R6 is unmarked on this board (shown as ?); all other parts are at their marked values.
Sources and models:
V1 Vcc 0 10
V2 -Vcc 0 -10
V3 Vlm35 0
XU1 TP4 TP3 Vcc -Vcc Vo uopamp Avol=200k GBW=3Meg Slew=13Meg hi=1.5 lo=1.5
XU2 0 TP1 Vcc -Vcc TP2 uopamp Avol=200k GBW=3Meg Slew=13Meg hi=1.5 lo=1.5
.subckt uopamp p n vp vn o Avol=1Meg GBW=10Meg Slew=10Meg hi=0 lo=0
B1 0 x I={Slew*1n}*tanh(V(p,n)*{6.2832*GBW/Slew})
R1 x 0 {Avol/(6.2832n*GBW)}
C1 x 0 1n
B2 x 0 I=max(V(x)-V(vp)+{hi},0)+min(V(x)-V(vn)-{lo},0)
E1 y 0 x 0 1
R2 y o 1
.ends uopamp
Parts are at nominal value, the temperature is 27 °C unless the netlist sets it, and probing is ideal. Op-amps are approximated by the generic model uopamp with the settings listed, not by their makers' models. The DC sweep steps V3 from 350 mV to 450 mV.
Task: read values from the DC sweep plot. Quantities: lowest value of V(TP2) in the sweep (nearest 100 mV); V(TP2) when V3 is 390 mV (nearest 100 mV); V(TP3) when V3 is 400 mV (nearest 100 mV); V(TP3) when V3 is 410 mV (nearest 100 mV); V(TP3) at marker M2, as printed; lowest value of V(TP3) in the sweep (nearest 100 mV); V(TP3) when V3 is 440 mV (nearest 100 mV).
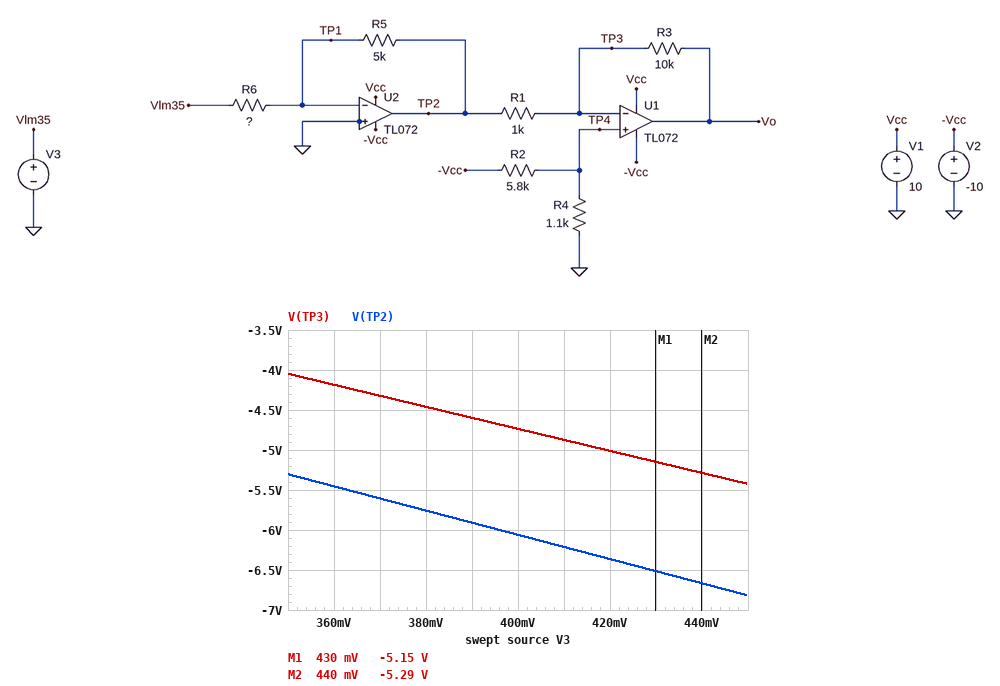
-6.8 V
-5.9 V
-4.7 V
-4.9 V
-5.29 V
-5.4 V
-5.3 V
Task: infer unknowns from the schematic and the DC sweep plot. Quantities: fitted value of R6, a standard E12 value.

330 Ω
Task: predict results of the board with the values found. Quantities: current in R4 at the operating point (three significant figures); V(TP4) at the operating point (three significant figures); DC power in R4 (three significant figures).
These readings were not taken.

1.45 mA
-1.59 V
2.31 mW
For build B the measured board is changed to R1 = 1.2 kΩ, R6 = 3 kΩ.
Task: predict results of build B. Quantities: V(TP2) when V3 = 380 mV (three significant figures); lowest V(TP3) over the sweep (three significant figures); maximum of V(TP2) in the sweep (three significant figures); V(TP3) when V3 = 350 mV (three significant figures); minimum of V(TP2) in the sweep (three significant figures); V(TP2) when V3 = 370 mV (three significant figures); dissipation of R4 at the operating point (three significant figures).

-633 mV
-1.58 V
-583 mV
-1.43 V
-750 mV
-617 mV
2.31 mW
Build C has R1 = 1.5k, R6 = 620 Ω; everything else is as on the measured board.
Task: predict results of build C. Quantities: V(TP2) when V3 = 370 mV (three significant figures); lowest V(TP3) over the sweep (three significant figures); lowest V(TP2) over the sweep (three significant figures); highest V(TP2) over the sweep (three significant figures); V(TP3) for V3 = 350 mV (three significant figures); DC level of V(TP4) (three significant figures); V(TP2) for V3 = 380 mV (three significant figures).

-2.98 V
-2.05 V
-3.63 V
-2.82 V
-1.59 V
-1.59 V
-3.06 V
